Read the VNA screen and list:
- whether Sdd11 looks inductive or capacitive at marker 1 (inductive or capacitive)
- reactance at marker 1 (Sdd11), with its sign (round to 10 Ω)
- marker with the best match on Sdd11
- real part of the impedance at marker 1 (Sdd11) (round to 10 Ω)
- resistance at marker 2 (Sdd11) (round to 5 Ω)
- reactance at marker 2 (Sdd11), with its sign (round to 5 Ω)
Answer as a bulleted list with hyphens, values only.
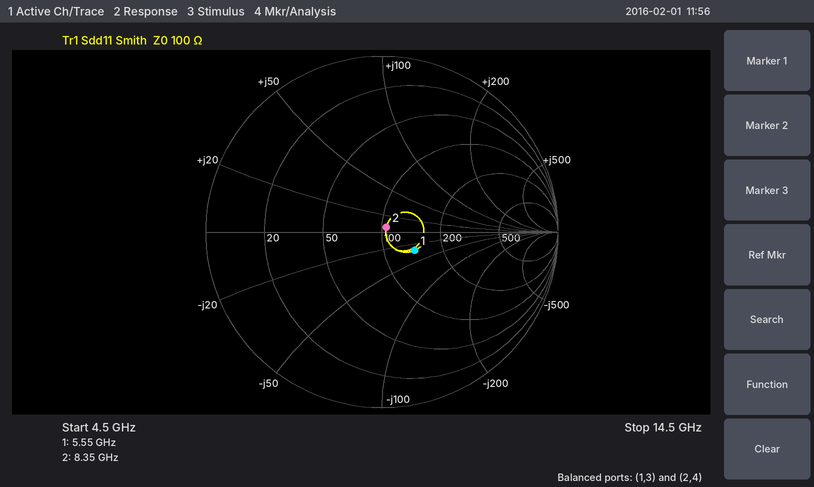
- capacitive
- -30 Ω
- marker 2
- 140 Ω
- 105 Ω
- +5 Ω
